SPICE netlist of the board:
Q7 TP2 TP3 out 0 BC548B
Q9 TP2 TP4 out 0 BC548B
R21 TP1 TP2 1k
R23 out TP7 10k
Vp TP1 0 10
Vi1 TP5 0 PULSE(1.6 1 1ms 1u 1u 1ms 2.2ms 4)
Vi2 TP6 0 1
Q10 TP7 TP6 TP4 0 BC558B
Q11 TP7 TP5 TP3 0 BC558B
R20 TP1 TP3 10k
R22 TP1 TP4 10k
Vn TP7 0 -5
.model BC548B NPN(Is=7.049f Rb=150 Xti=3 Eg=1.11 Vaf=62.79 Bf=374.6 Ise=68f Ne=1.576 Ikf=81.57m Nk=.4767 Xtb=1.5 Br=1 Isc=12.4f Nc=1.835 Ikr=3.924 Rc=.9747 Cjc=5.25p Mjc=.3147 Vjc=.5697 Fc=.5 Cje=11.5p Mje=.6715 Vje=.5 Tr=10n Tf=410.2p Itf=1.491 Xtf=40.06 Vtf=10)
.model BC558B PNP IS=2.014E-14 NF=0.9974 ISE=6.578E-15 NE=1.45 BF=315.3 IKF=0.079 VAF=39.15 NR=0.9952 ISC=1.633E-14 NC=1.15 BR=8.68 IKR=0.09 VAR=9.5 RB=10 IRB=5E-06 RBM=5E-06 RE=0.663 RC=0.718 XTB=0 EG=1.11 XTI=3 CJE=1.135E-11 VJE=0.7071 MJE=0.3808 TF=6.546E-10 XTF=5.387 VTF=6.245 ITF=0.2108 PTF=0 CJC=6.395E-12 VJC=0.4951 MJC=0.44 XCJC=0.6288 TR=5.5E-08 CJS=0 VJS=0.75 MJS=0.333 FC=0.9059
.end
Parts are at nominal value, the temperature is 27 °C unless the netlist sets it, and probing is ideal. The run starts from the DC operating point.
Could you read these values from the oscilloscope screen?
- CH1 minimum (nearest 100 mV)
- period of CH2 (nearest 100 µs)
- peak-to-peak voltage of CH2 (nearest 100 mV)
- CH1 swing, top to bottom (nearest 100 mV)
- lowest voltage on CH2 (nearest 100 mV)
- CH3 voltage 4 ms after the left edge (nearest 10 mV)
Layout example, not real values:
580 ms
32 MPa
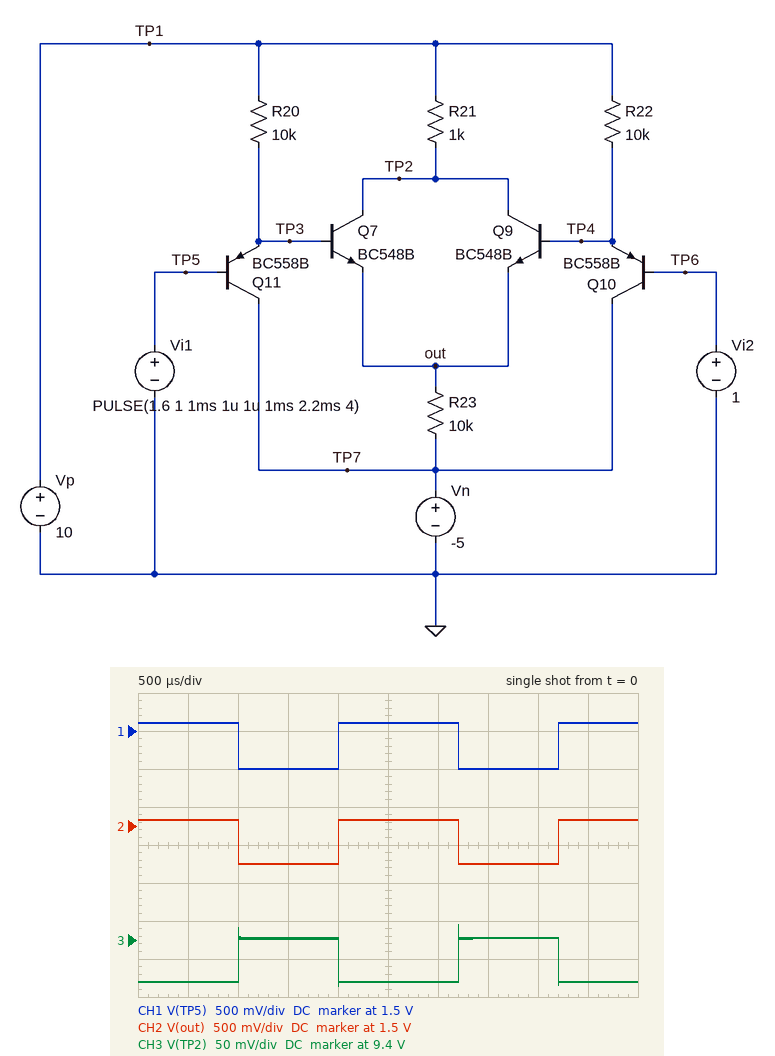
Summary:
1.0 V
2.2 ms
600 mV
600 mV
1.0 V
9.40 V
